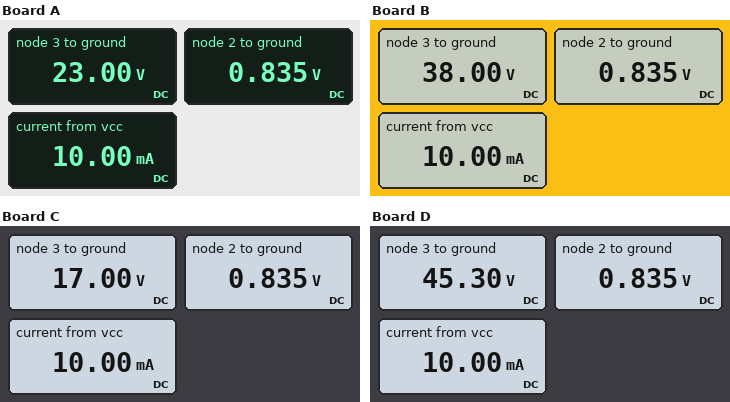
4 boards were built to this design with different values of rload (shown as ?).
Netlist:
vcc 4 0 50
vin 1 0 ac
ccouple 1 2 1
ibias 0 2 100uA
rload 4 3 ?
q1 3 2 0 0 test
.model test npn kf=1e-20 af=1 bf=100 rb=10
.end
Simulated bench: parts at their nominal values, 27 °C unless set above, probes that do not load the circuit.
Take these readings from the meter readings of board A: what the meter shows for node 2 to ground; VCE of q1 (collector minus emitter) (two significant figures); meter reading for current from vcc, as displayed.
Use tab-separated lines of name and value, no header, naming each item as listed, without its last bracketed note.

what the meter shows for node 2 to ground	0.835 V
VCE of q1 (collector minus emitter)	23 V
meter reading for current from vcc, as displayed	10.00 mA
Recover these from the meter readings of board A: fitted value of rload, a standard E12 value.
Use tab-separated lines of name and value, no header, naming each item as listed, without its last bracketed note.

fitted value of rload, a standard E12 value	2.7 kΩ
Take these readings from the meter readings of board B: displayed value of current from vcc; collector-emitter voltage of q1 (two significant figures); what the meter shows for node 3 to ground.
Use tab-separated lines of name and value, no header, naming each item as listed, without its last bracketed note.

displayed value of current from vcc	10.00 mA
collector-emitter voltage of q1	38 V
what the meter shows for node 3 to ground	38.00 V
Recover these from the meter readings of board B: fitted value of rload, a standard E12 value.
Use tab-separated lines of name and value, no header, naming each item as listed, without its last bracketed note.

fitted value of rload, a standard E12 value	1.2 kΩ
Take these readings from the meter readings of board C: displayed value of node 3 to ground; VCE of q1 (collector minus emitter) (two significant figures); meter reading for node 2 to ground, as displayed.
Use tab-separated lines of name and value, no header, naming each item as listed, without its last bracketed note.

displayed value of node 3 to ground	17.00 V
VCE of q1 (collector minus emitter)	17 V
meter reading for node 2 to ground, as displayed	0.835 V
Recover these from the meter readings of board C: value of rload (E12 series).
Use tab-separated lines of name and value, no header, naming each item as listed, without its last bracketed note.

value of rload	3.3 kΩ
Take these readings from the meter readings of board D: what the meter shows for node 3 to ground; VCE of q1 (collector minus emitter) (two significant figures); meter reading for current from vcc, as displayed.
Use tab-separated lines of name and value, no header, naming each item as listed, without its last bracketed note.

what the meter shows for node 3 to ground	45.30 V
VCE of q1 (collector minus emitter)	45 V
meter reading for current from vcc, as displayed	10.00 mA
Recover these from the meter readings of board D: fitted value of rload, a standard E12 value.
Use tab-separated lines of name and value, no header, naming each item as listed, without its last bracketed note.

fitted value of rload, a standard E12 value	470 Ω
